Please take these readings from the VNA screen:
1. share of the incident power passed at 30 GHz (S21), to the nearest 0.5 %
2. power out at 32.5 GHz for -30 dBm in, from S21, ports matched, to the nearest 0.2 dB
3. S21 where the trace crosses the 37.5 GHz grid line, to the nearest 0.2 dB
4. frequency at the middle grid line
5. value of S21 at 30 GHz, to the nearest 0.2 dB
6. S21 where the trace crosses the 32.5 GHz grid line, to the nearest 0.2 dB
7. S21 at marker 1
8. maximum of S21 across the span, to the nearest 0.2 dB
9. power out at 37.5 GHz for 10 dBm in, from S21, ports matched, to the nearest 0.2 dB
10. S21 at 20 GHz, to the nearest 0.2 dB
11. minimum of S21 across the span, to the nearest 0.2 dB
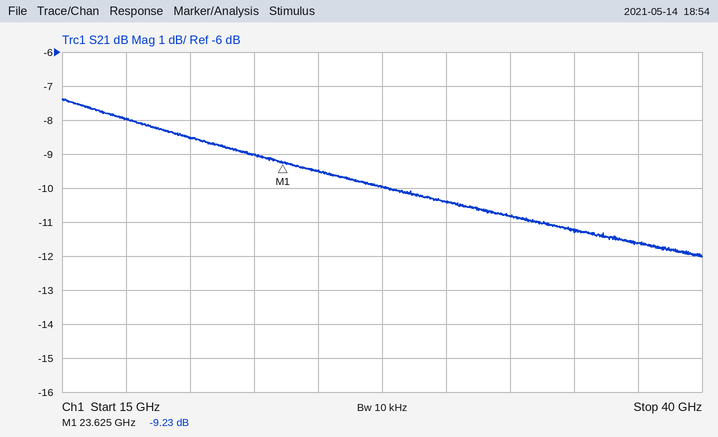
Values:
9.0 %
-40.8 dBm
-11.6 dB
27.5 GHz
-10.4 dB
-10.8 dB
-9.23 dB
-7.4 dB
-1.6 dBm
-8.6 dB
-12.0 dB
